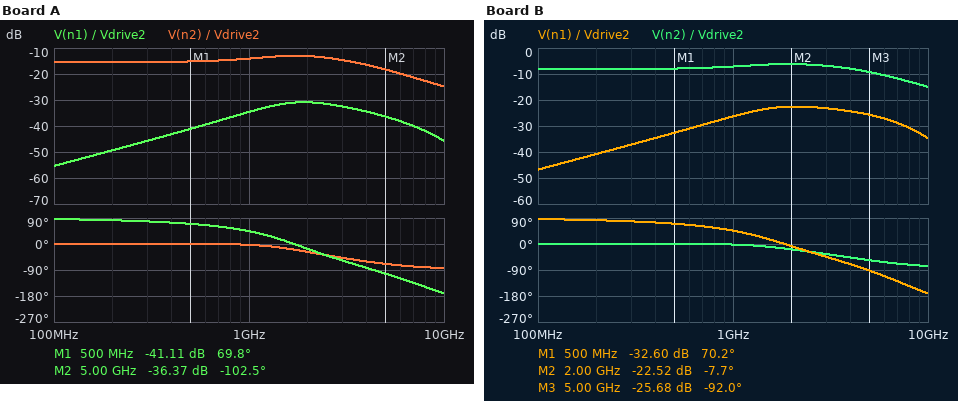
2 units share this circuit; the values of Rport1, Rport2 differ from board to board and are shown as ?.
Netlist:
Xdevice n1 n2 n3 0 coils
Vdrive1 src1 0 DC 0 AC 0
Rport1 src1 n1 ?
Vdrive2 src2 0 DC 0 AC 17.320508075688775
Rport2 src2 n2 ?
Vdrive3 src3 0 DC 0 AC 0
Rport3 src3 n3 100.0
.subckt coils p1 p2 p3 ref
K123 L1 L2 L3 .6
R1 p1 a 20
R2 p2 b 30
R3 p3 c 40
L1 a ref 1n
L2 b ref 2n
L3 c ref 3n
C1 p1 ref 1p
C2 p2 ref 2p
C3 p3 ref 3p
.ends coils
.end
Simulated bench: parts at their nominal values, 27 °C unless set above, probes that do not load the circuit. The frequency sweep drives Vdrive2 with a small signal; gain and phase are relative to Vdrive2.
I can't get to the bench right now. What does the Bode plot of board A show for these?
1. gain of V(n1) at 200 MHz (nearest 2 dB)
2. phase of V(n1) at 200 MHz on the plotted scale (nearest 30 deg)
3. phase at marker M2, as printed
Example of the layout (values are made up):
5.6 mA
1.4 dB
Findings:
-50 dB
90 deg
-102.5 deg
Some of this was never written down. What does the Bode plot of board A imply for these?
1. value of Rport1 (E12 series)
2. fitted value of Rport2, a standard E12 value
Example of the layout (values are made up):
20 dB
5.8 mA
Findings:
27 Ω
150 Ω
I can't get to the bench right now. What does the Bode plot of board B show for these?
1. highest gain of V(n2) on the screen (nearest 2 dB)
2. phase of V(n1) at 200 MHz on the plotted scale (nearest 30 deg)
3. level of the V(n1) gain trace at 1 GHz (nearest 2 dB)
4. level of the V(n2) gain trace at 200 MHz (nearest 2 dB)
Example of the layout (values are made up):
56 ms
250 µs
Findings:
-6 dB
90 deg
-26 dB
-8 dB
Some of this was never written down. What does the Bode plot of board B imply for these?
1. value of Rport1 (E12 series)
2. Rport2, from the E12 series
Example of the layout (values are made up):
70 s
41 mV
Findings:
39 Ω
47 Ω
